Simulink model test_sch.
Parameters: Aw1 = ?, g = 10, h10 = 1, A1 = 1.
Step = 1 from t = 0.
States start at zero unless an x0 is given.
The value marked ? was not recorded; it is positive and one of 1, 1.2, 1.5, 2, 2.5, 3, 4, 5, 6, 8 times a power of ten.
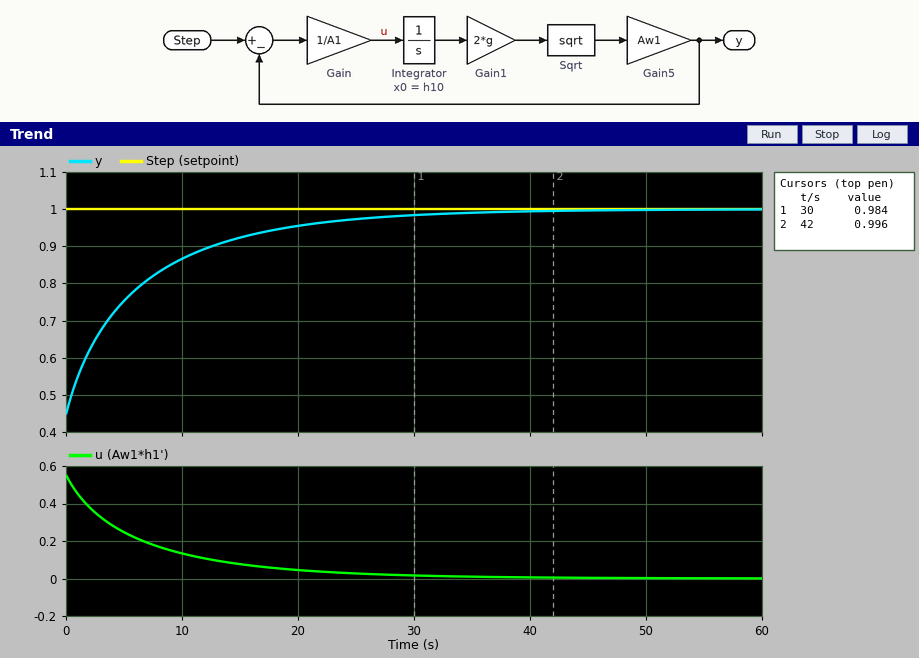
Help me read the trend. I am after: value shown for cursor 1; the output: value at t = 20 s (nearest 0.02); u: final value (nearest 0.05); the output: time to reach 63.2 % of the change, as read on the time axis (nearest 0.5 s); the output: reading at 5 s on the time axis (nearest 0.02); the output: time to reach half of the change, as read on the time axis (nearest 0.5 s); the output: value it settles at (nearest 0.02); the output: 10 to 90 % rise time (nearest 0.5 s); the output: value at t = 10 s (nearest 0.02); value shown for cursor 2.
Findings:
0.984
0.96
0.00
6.5 s
0.76
4.0 s
1.00
17.5 s
0.86
0.996
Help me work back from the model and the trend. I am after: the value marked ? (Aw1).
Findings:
0.1
